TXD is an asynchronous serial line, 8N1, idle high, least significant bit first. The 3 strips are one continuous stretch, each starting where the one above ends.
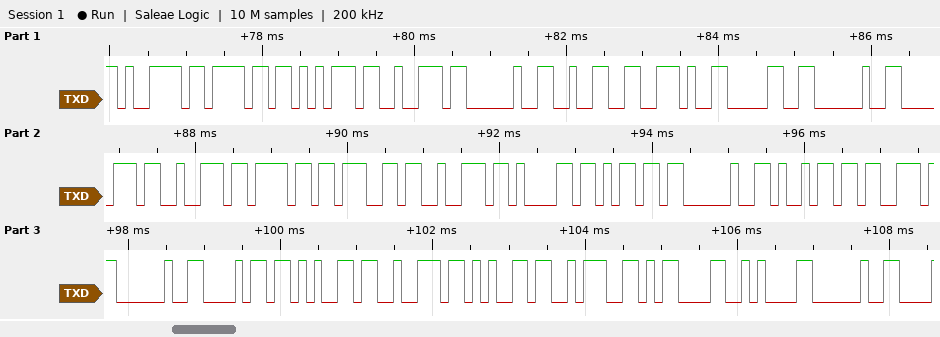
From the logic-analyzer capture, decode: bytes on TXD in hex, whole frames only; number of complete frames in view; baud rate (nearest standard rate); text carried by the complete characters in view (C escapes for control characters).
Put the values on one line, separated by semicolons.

79 6F 75 72 20 32 2E 30 20 70 72 6F 67 72 61 6D 20 69 73 20 68 65 72 65 3A 0D 0A 20; 28; 9600 baud; "your 2.0 program is here:\r\n "
